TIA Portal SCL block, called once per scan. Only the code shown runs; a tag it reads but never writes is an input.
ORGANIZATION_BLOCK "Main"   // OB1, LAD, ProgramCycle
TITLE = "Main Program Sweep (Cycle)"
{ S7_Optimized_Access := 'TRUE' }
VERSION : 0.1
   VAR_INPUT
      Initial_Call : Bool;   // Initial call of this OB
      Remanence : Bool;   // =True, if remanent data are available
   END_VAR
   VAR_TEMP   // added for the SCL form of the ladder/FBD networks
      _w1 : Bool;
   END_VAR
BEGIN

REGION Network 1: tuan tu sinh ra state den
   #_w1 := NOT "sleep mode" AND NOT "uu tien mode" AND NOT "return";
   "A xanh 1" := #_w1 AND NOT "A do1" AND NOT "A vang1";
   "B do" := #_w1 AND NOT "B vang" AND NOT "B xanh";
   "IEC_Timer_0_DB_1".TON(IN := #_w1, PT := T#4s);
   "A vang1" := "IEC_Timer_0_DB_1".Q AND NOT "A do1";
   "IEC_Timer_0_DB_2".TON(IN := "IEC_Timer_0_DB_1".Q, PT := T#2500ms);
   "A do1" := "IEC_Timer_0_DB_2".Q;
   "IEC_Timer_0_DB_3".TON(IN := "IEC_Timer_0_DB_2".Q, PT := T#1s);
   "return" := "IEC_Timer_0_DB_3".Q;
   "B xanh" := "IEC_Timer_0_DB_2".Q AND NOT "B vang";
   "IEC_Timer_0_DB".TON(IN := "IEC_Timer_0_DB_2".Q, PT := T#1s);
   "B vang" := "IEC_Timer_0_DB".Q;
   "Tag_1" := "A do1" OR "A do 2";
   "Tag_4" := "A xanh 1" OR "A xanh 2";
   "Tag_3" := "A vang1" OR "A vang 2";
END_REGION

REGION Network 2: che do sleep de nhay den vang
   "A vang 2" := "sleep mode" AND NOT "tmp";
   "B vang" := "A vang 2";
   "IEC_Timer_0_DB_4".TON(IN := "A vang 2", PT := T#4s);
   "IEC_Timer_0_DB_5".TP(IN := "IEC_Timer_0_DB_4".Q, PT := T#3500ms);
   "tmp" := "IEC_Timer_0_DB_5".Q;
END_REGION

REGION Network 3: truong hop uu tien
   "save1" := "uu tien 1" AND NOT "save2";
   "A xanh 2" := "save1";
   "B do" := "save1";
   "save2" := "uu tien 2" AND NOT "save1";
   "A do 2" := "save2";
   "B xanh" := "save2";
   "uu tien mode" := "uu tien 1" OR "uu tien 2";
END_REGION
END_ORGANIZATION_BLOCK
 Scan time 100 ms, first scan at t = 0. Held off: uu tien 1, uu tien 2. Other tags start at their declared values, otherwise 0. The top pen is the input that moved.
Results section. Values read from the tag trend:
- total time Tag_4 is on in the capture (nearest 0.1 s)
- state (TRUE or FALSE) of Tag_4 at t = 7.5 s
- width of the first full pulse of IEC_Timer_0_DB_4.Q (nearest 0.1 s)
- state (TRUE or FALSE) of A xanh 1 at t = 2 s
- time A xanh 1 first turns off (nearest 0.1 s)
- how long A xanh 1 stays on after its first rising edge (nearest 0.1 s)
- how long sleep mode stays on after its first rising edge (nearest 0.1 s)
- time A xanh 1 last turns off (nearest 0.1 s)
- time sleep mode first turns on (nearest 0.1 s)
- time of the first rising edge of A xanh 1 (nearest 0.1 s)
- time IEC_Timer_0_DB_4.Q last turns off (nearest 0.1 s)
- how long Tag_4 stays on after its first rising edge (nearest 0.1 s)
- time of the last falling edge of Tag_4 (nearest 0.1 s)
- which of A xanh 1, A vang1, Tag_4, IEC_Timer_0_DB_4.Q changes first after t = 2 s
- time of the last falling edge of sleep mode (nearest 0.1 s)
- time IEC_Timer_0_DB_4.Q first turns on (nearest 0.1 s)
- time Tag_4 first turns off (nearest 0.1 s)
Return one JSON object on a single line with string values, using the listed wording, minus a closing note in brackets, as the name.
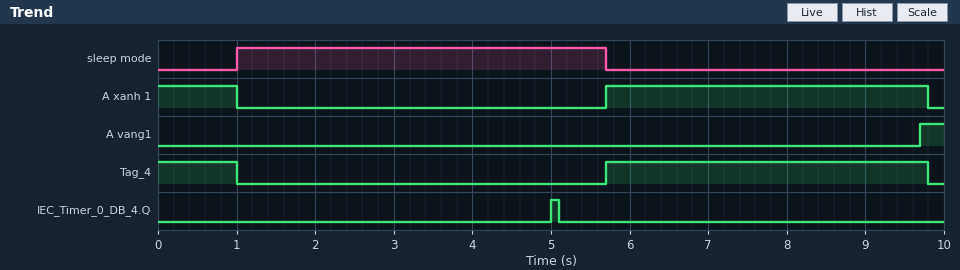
{"total time Tag_4 is on in the capture": "5.1 s", "state (TRUE or FALSE) of Tag_4 at t = 7.5 s": "TRUE", "width of the first full pulse of IEC_Timer_0_DB_4.Q": "0.1 s", "state (TRUE or FALSE) of A xanh 1 at t = 2 s": "FALSE", "time A xanh 1 first turns off": "1.0 s", "how long A xanh 1 stays on after its first rising edge": "4.1 s", "how long sleep mode stays on after its first rising edge": "4.7 s", "time A xanh 1 last turns off": "9.8 s", "time sleep mode first turns on": "1.0 s", "time of the first rising edge of A xanh 1": "5.7 s", "time IEC_Timer_0_DB_4.Q last turns off": "5.1 s", "how long Tag_4 stays on after its first rising edge": "4.1 s", "time of the last falling edge of Tag_4": "9.8 s", "which of A xanh 1, A vang1, Tag_4, IEC_Timer_0_DB_4.Q changes first after t = 2 s": "IEC_Timer_0_DB_4.Q", "time of the last falling edge of sleep mode": "5.7 s", "time IEC_Timer_0_DB_4.Q first turns on": "5.0 s", "time Tag_4 first turns off": "1.0 s"}
